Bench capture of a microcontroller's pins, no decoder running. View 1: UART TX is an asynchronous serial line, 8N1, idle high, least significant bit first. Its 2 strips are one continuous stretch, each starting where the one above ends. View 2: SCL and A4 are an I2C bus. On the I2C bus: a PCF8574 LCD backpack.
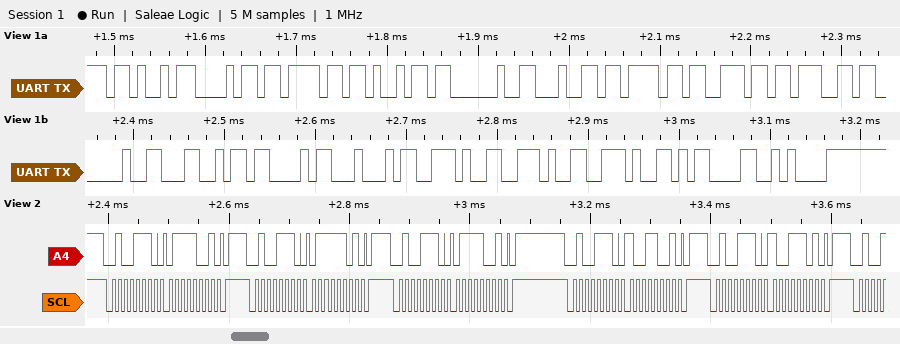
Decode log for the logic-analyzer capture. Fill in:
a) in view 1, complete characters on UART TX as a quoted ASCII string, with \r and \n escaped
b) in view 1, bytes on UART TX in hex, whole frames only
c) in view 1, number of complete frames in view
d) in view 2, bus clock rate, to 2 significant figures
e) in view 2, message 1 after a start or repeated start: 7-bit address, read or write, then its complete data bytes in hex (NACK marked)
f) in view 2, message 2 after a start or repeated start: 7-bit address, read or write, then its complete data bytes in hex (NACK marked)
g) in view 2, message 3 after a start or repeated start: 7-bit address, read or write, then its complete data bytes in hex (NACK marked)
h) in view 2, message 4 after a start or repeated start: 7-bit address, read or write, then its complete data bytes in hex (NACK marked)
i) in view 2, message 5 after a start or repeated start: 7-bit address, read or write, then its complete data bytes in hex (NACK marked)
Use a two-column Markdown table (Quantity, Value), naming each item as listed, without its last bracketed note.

| Quantity | Value |
|---|---|
| in view 1, complete characters on UART TX as a quoted ASCII string, with \r and \n escaped | "Khoi dong LCD...\r\n" |
| in view 1, bytes on UART TX in hex, whole frames only | 0x4B 0x68 0x6F 0x69 0x20 0x64 0x6F 0x6E 0x67 0x20 0x4C 0x43 0x44 0x2E 0x2E 0x2E 0x0D 0x0A |
| in view 1, number of complete frames in view | 18 |
| in view 2, bus clock rate, to 2 significant figures | 100 kHz |
| in view 2, message 1 after a start or repeated start: 7-bit address, read or write, then its complete data bytes in hex | 0x27 write: 79 |
| in view 2, message 2 after a start or repeated start: 7-bit address, read or write, then its complete data bytes in hex | 0x27 write: 7D |
| in view 2, message 3 after a start or repeated start: 7-bit address, read or write, then its complete data bytes in hex | 0x27 write: 79 |
| in view 2, message 4 after a start or repeated start: 7-bit address, read or write, then its complete data bytes in hex | 0x27 write: 99 |
| in view 2, message 5 after a start or repeated start: 7-bit address, read or write, then its complete data bytes in hex | 0x27 write: 9D |
